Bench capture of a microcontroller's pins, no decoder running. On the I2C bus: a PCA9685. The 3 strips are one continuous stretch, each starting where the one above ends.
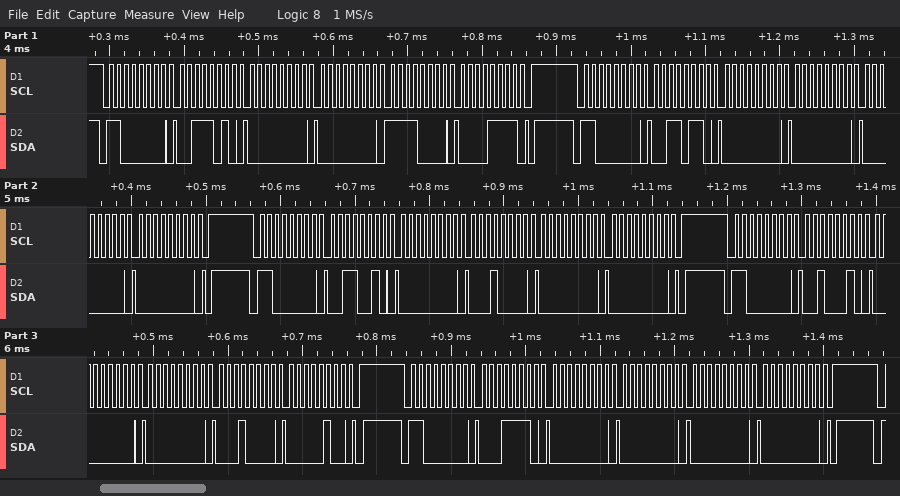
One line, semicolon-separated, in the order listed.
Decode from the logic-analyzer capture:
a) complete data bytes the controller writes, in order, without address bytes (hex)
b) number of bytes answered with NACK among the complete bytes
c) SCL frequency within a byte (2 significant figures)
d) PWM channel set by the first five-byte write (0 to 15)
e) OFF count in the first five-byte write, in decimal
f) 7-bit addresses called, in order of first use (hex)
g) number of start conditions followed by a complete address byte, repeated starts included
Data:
3A 00 00 F0 0F 36 00 00 00 00 32 00 10 00 00 22 00 00 10 04 1E 00 00 00 00; 0; 100 kHz; 13; 4080; 0x60; 5
